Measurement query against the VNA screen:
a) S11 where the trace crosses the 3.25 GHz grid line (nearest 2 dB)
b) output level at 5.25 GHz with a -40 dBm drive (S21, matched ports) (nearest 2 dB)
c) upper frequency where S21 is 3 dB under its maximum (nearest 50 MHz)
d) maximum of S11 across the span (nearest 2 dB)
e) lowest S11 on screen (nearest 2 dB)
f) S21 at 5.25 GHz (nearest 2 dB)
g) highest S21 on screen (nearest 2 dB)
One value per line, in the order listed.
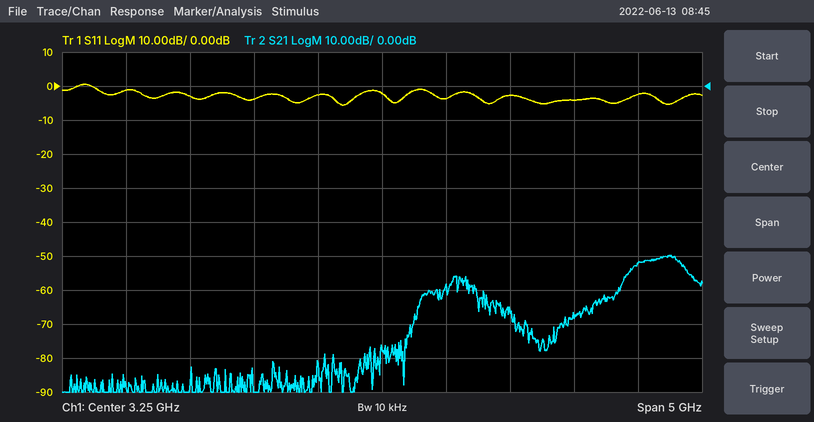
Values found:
-2 dB
-92 dBm
5.60 GHz
0 dB
-6 dB
-52 dB
-50 dB
